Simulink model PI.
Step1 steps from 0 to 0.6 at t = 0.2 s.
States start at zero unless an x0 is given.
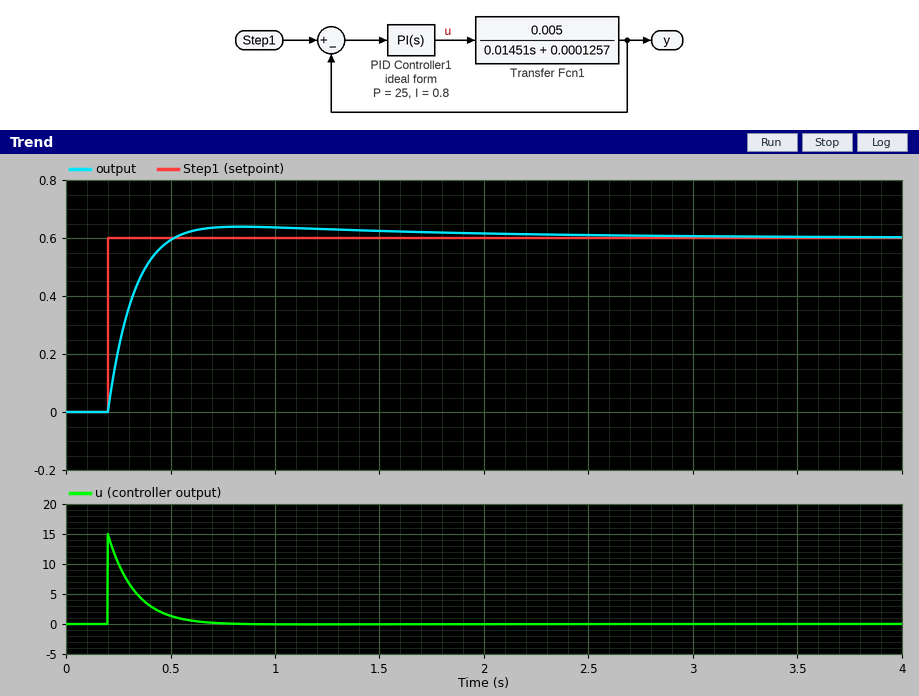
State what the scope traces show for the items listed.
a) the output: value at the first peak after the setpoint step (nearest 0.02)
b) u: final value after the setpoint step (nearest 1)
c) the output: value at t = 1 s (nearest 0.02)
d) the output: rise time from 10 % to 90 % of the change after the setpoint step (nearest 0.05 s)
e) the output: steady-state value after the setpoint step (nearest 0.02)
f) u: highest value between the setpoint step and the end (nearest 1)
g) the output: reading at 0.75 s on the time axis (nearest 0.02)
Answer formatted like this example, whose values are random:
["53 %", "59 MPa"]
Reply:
["0.64", "0", "0.64", "0.20 s", "0.60", "15", "0.64"]
